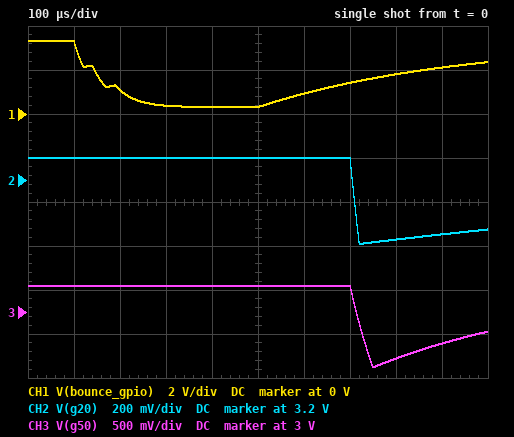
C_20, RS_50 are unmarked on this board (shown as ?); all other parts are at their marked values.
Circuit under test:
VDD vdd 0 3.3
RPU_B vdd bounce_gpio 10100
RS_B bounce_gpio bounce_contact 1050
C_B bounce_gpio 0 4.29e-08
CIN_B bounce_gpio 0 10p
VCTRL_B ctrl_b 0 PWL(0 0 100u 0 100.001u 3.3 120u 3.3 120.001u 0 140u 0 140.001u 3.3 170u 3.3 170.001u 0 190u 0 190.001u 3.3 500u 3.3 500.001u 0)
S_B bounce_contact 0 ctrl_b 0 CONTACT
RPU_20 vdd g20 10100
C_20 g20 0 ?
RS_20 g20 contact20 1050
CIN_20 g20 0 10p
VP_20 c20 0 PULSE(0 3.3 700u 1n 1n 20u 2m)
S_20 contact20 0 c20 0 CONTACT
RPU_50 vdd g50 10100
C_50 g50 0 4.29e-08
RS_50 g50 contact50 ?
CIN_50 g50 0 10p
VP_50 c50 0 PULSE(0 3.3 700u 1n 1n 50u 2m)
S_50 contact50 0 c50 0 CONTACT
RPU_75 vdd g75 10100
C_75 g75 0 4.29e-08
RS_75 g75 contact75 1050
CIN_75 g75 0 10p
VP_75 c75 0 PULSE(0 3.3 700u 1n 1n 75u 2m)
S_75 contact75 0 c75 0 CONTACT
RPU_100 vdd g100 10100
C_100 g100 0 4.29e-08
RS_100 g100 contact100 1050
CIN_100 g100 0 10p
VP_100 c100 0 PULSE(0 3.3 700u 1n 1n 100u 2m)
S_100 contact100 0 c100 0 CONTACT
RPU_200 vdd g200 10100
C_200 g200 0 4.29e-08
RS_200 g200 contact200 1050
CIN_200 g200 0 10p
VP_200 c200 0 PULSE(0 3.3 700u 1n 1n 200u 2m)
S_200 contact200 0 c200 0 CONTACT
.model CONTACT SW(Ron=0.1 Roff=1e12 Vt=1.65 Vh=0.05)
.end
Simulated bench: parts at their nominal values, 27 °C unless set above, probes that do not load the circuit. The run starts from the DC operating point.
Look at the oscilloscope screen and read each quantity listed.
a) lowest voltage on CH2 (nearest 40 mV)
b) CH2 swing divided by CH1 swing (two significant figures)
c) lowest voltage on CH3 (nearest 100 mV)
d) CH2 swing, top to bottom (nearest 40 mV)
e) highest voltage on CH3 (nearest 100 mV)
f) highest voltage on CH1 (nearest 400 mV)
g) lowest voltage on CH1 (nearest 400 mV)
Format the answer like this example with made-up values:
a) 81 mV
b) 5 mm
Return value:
a) 2.92 V
b) 0.13
c) 2.4 V
d) 400 mV
e) 3.3 V
f) 3.2 V
g) 400 mV
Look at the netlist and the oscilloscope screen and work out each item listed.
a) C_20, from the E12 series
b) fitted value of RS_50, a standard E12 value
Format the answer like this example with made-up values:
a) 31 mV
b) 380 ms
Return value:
a) 150 nF
b) 3.3 kΩ
